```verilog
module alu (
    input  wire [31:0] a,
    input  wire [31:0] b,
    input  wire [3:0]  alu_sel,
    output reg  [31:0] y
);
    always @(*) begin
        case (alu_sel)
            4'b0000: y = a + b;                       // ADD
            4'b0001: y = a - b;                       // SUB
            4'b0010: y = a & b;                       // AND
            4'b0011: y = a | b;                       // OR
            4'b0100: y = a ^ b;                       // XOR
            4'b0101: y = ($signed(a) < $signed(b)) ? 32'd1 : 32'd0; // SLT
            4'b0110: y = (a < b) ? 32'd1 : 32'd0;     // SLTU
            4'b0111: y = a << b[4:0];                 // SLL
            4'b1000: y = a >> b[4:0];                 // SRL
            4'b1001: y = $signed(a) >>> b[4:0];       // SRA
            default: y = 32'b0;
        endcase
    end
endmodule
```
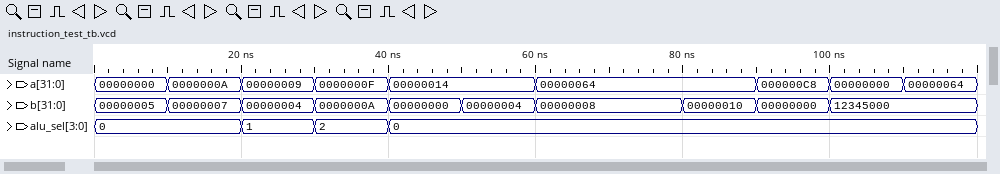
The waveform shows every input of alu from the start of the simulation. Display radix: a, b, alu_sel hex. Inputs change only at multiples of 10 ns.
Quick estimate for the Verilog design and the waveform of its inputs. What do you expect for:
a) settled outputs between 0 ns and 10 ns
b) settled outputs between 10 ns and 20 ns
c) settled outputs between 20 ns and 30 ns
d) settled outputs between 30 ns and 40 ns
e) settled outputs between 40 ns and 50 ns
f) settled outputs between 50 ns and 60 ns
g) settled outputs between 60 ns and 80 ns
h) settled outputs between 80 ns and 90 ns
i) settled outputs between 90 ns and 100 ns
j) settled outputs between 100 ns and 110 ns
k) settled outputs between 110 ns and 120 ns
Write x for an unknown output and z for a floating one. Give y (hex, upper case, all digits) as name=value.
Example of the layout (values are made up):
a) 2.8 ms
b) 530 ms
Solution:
a) y=00000005
b) y=00000011
c) y=00000005
d) y=0000000A
e) y=00000014
f) y=00000018
g) y=0000006C
h) y=00000074
i) y=000000C8
j) y=12345000
k) y=12345064
